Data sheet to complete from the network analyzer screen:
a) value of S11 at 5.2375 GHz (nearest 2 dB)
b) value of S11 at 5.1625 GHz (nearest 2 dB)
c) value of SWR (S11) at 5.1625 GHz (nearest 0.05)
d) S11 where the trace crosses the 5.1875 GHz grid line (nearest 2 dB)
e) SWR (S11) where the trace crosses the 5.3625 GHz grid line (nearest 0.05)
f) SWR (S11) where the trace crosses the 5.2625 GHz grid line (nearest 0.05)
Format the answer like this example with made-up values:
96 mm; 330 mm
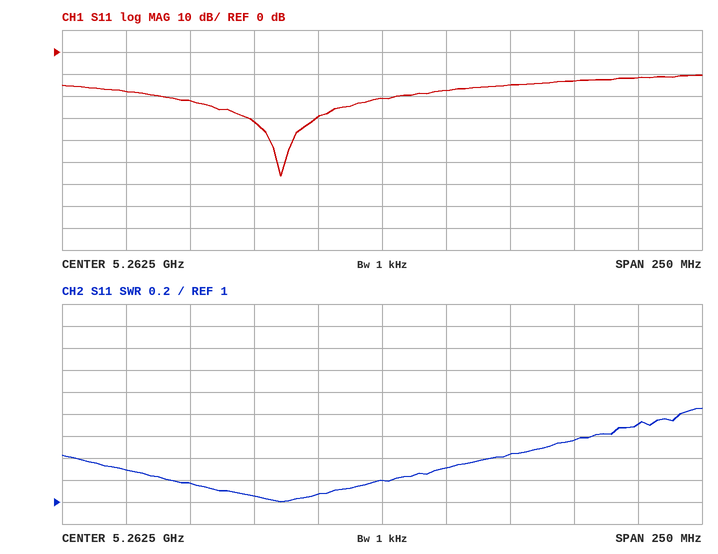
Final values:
-30 dB; -18 dB; 1.30; -22 dB; 1.70; 1.20
